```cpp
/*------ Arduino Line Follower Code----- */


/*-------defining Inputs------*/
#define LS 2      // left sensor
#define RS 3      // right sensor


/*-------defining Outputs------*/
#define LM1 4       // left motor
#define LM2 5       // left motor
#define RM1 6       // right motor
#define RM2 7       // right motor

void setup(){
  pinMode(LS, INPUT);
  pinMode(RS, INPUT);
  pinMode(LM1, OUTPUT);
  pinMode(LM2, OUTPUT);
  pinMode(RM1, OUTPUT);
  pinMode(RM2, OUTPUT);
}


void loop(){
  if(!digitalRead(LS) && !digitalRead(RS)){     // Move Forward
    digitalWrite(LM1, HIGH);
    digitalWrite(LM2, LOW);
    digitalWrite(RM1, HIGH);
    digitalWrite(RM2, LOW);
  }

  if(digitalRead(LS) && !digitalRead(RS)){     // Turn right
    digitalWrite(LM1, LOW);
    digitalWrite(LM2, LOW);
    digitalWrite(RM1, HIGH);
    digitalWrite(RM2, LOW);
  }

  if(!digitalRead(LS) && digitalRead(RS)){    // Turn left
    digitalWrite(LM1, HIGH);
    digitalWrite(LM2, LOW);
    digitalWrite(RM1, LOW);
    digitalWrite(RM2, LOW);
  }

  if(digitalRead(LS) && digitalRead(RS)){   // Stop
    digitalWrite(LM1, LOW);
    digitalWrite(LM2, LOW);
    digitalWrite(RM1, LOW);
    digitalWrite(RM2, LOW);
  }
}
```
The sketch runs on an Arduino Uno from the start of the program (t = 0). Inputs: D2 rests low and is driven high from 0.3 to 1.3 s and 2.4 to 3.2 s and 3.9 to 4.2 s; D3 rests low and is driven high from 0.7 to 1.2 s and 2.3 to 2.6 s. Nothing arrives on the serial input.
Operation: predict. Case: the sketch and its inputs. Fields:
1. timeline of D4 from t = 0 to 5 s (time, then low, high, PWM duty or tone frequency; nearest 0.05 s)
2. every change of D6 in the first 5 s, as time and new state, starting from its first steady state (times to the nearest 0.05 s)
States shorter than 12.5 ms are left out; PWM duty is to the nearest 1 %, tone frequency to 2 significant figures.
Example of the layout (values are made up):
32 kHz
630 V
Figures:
0 s high; 0.3 s low; 1.3 s high; 2.4 s low; 3.2 s high; 3.9 s low; 4.2 s high
0 s high; 0.7 s low; 1.2 s high; 2.3 s low; 2.6 s high
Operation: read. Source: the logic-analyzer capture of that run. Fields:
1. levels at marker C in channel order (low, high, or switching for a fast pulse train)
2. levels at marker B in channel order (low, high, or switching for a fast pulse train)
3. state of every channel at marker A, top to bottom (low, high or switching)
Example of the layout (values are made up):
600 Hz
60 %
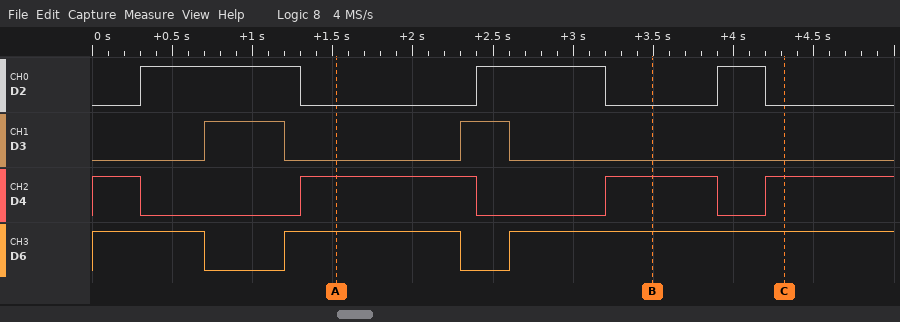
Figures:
D2 low, D3 low, D4 high, D6 high
D2 low, D3 low, D4 high, D6 high
D2 low, D3 low, D4 high, D6 high
